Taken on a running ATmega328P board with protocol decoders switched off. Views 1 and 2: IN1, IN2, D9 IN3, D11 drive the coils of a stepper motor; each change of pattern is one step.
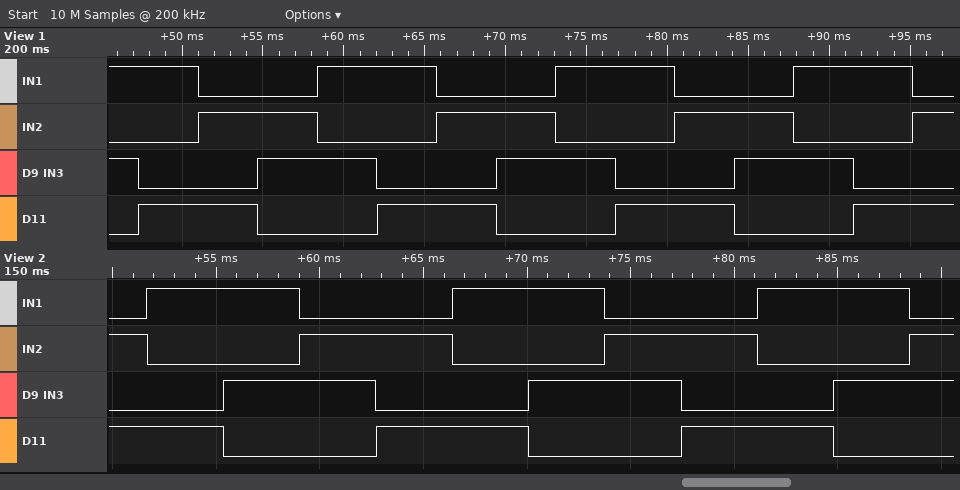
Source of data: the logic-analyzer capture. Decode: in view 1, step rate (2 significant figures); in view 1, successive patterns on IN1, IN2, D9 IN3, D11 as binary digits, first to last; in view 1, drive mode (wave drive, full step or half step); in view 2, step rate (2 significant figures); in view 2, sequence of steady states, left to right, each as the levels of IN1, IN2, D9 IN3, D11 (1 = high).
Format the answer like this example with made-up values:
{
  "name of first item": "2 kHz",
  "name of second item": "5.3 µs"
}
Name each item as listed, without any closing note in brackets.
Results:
{
  "in view 1, step rate": "270 steps/s",
  "in view 1, successive patterns on IN1, IN2, D9 IN3, D11 as binary digits, first to last": "1010 1001 0101 0110 1010 1001 0101 0110 1010 1001 0101 0110 1010 1001 0101",
  "in view 1, drive mode": "full step",
  "in view 2, step rate": "270 steps/s",
  "in view 2, sequence of steady states, left to right, each as the levels of IN1, IN2, D9 IN3, D11": "0101 1001 1010 0110 0101 1001 1010 0110 0101 1001 1010 0110"
}
